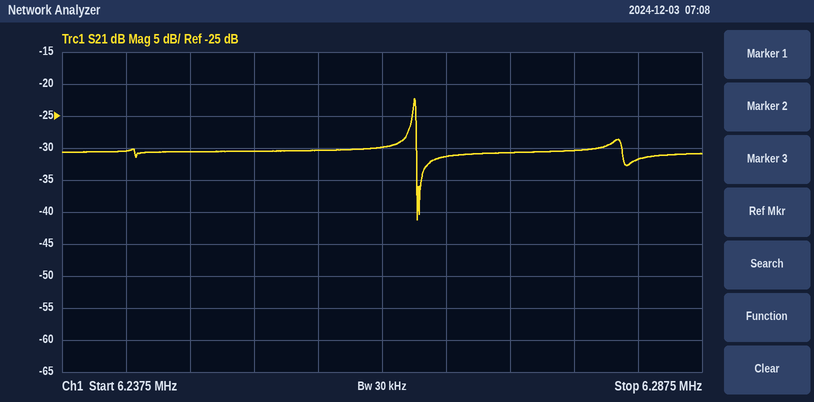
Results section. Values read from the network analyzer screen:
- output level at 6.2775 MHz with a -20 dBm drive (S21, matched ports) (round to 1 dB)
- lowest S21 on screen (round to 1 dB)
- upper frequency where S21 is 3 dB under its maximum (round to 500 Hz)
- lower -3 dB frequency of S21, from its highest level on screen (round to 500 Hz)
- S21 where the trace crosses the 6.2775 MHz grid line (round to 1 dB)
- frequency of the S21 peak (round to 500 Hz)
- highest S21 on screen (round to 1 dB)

-50 dBm
-41 dB
6.2650 MHz
6.2650 MHz
-30 dB
6.2650 MHz
-22 dB
